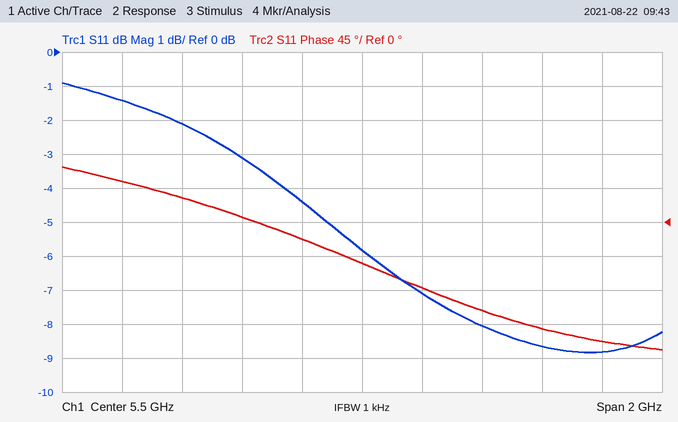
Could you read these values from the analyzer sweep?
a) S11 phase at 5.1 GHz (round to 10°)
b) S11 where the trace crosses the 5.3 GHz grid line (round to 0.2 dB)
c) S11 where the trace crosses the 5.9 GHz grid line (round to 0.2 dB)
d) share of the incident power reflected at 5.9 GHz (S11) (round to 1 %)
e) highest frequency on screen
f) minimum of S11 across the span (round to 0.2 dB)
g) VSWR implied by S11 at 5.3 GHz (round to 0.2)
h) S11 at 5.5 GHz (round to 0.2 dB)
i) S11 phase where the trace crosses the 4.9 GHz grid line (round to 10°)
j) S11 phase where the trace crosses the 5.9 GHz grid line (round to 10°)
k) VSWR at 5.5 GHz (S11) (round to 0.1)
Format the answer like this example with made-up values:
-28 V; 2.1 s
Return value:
10°; -4.4 dB; -8.0 dB; 16 %; 6.5 GHz; -8.8 dB; 4.0; -5.8 dB; 30°; -120°; 3.1
